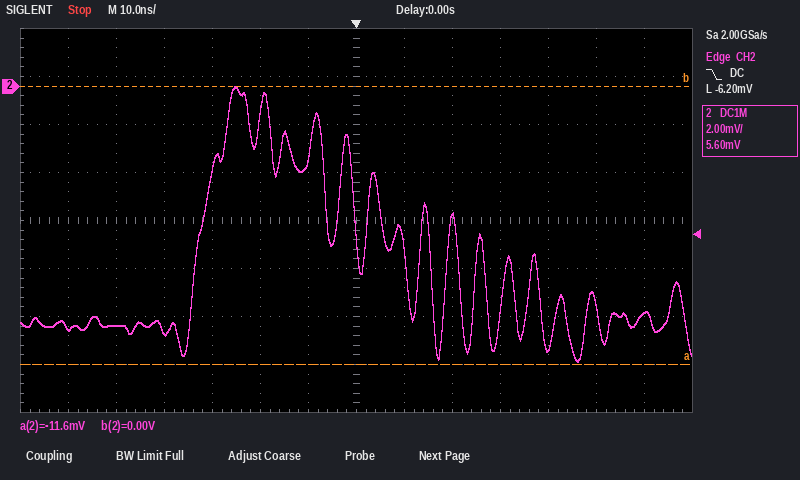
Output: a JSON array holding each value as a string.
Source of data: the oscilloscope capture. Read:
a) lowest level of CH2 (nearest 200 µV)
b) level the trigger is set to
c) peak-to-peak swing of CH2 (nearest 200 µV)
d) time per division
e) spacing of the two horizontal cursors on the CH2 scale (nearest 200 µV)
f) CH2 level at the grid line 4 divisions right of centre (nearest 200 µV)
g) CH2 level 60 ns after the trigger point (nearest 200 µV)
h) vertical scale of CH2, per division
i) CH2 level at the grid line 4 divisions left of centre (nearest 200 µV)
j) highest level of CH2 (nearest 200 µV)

["-11.4 mV", "-6.20 mV", "11.4 mV", "10 ns", "11.6 mV", "-11.0 mV", "-9.4 mV", "2 mV", "-10.2 mV", "0.0 mV"]
